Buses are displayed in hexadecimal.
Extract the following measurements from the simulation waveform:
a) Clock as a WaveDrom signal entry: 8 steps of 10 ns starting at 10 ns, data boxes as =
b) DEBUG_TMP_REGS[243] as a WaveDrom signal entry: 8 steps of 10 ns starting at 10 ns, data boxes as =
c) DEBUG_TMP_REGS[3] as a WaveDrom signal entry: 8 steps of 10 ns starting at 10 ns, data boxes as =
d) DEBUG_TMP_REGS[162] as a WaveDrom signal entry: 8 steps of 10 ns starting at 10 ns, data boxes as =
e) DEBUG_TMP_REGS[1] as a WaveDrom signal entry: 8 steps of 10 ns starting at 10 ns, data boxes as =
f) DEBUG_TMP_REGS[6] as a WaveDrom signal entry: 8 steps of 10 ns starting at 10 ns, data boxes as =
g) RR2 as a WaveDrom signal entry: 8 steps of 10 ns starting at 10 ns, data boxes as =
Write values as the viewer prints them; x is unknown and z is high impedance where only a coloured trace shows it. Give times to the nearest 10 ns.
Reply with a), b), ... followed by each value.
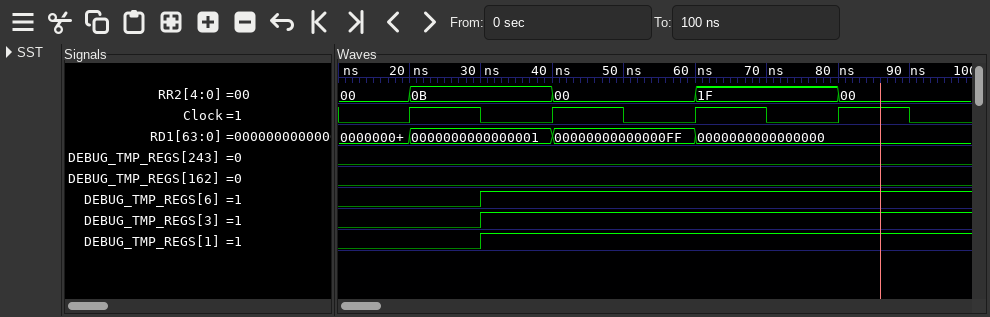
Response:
a) {name: 'Clock', wave: '01010101'}
b) {name: 'DEBUG_TMP_REGS[243]', wave: '0.......'}
c) {name: 'DEBUG_TMP_REGS[3]', wave: '0.1.....'}
d) {name: 'DEBUG_TMP_REGS[162]', wave: '0.......'}
e) {name: 'DEBUG_TMP_REGS[1]', wave: '0.1.....'}
f) {name: 'DEBUG_TMP_REGS[6]', wave: '0.1.....'}
g) {name: 'RR2', wave: '==.=.=.=', data: '00 0B 00 1F 00'}
